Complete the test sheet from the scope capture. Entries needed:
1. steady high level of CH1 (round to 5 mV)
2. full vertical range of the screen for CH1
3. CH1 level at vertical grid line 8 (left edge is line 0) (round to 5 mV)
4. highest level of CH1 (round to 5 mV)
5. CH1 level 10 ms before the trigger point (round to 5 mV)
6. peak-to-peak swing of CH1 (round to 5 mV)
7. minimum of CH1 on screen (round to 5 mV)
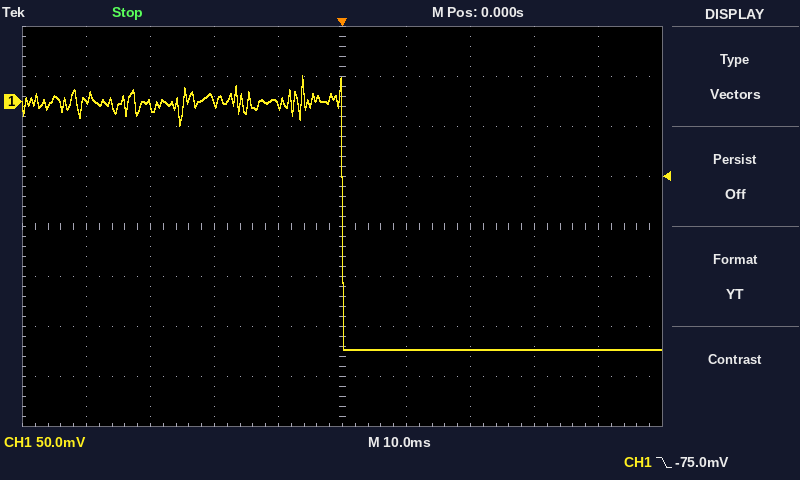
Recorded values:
0 mV
400 mV
-250 mV
25 mV
-5 mV
275 mV
-250 mV
